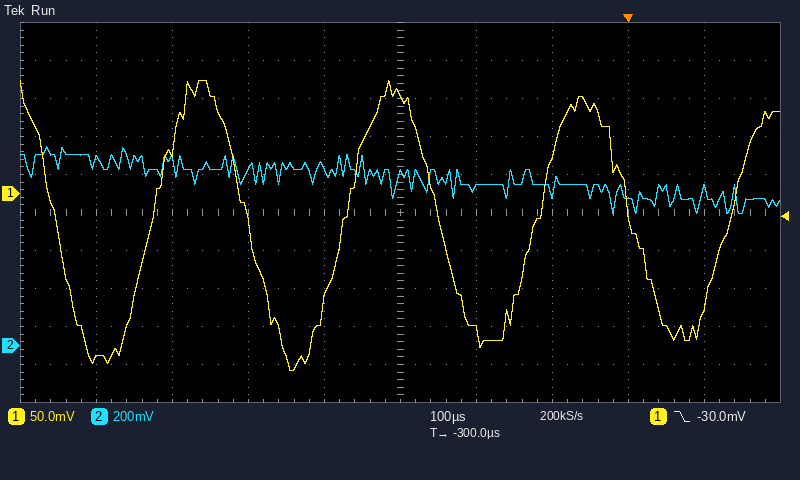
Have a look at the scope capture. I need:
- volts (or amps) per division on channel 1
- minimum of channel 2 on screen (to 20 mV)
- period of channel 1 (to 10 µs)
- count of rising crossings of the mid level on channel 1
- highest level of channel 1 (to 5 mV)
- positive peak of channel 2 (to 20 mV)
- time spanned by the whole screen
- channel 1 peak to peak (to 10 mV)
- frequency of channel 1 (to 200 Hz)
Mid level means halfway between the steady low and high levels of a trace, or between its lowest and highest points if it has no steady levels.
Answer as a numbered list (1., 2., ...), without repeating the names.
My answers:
1. 50 mV
2. 700 mV
3. 250 µs
4. 4
5. 150 mV
6. 1.04 V
7. 1 ms
8. 380 mV
9. 4.0 kHz
